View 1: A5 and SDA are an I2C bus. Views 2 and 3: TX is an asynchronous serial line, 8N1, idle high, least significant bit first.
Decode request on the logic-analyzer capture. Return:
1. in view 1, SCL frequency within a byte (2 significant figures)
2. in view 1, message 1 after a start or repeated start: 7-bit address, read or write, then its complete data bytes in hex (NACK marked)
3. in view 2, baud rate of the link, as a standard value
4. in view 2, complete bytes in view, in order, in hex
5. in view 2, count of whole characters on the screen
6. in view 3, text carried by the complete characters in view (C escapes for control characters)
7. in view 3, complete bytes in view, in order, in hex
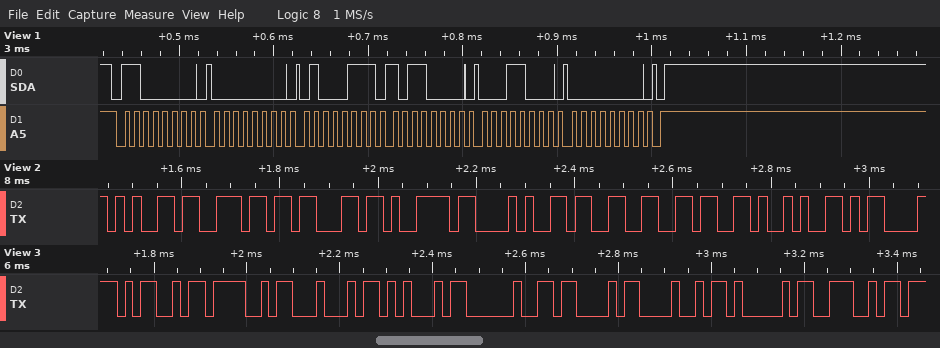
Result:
100 kHz
0x60 write: 00 47 B0 18 00
57600 baud
0x65 0x6E 0x63 0x79 0x28 0x33 0x36 0x29 0x0D
9
"MODE CHAN"
4D 4F 44 45 20 43 48 41 4E
